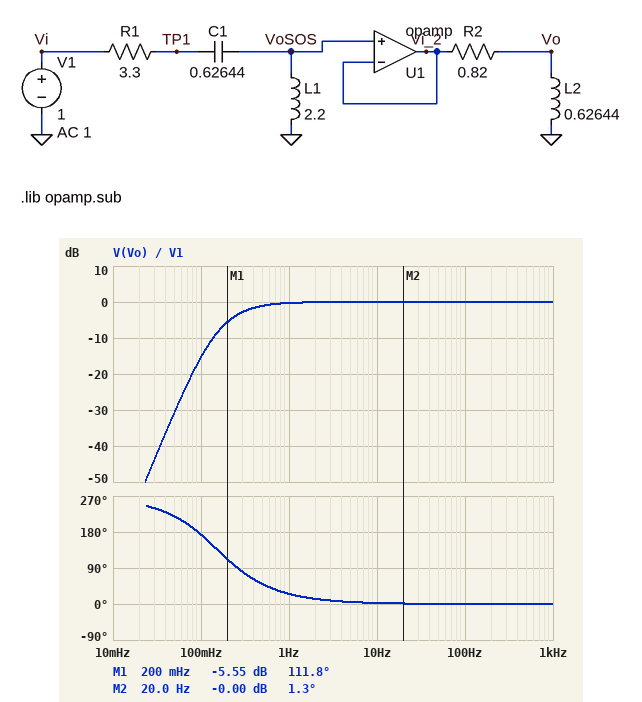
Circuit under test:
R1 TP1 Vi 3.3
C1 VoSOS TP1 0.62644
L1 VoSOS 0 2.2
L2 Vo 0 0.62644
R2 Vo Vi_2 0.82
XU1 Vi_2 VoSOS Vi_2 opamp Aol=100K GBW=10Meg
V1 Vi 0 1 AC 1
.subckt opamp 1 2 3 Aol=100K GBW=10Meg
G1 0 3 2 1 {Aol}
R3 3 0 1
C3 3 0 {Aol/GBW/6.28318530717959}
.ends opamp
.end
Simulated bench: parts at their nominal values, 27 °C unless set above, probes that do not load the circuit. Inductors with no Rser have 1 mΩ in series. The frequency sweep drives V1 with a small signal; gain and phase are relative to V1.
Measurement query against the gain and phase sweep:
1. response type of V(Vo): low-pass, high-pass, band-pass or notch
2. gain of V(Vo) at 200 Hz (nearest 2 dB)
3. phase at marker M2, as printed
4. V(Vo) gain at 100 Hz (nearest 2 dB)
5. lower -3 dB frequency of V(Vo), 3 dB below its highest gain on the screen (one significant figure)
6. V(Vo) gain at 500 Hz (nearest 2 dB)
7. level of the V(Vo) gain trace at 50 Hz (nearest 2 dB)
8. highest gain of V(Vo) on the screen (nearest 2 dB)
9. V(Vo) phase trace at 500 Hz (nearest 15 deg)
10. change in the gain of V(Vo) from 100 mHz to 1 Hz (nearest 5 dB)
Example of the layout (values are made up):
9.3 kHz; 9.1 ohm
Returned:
high-pass; 0 dB; 1.3 deg; 0 dB; 300 mHz; 0 dB; 0 dB; 0 dB; 0 deg; 15 dB
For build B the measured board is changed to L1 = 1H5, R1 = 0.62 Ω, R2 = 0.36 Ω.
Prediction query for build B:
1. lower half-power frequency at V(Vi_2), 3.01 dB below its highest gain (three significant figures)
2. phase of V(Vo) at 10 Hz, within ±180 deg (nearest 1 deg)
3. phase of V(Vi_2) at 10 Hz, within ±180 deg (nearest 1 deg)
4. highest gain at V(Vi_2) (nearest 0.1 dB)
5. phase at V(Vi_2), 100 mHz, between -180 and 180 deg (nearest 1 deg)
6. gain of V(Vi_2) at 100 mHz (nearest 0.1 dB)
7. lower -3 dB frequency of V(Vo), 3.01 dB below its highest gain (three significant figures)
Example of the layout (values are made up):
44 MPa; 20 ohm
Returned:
143 mHz; 1 deg; 0 deg; 8.1 dB; 159 deg; -5.2 dB; 145 mHz
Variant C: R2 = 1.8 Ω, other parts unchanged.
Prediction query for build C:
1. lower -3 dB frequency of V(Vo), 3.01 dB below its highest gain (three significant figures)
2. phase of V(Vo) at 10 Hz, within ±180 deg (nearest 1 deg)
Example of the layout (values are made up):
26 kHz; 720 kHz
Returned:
499 mHz; 4 deg
